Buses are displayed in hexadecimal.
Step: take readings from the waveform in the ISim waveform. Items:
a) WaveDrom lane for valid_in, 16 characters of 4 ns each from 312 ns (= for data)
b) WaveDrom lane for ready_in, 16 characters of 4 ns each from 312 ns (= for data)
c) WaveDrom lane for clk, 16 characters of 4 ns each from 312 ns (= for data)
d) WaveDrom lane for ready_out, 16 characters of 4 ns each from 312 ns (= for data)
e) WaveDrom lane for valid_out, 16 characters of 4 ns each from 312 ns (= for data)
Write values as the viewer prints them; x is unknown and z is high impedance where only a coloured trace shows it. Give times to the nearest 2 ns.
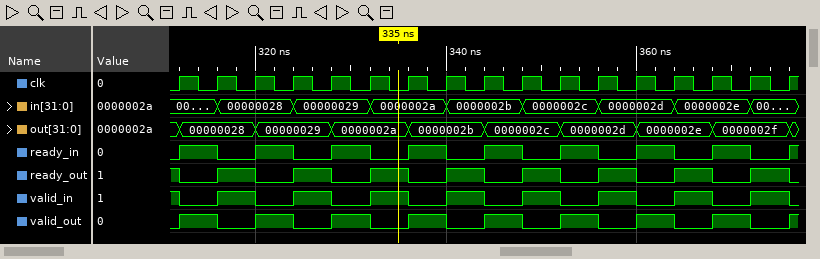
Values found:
{name: 'valid_in', wave: '0101010101010101'}
{name: 'ready_in', wave: '1010101010101010'}
{name: 'clk', wave: 'p...............'}
{name: 'ready_out', wave: '0101010101010101'}
{name: 'valid_out', wave: '1010101010101010'}
